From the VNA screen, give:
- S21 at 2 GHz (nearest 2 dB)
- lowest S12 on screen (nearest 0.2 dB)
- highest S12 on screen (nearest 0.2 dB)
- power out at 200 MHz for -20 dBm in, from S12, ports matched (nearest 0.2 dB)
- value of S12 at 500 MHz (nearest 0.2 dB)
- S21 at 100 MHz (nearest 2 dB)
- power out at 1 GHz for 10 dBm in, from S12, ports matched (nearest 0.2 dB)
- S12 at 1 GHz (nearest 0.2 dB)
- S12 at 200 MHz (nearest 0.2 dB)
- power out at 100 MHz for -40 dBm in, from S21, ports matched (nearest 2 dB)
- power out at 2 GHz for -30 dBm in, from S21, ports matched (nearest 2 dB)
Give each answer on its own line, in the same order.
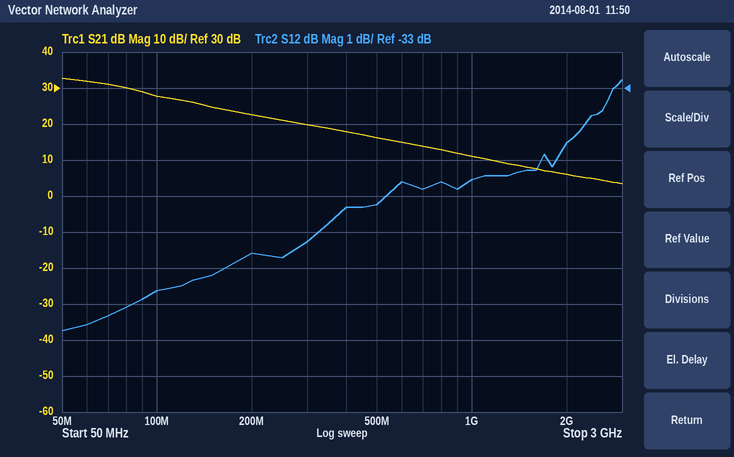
6 dB
-39.8 dB
-32.8 dB
-57.6 dBm
-36.2 dB
28 dB
-25.6 dBm
-35.6 dB
-37.6 dB
-12 dBm
-24 dBm
